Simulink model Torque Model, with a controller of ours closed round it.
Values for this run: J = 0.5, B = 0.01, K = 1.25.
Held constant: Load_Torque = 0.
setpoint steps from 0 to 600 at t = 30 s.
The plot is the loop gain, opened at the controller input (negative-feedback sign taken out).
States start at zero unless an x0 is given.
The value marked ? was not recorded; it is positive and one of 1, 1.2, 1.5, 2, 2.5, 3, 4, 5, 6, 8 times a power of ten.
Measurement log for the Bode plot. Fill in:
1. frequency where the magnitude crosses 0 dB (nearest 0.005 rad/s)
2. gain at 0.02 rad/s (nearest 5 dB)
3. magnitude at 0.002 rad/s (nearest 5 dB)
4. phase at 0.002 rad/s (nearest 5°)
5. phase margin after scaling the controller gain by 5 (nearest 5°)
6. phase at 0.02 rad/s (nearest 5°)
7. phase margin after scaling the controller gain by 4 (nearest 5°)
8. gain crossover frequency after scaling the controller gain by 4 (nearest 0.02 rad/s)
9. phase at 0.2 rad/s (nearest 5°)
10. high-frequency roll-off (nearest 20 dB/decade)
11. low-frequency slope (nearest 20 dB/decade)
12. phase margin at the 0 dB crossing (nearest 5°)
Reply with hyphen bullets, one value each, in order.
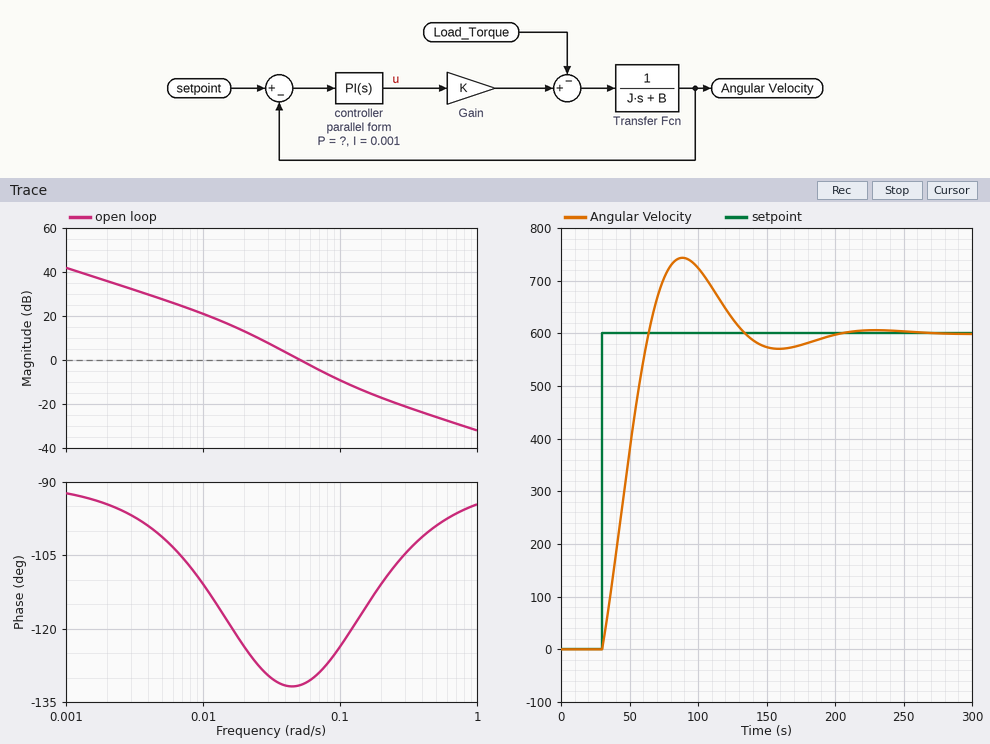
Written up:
- 0.050 rad/s
- 15 dB
- 35 dB
- -95°
- 65°
- -125°
- 60°
- 0.12 rad/s
- -110°
- -20 dB/decade
- -20 dB/decade
- 50°
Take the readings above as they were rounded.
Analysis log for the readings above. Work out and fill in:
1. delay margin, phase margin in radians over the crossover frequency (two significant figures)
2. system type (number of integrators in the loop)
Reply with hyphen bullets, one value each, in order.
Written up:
- 17 s
- 1
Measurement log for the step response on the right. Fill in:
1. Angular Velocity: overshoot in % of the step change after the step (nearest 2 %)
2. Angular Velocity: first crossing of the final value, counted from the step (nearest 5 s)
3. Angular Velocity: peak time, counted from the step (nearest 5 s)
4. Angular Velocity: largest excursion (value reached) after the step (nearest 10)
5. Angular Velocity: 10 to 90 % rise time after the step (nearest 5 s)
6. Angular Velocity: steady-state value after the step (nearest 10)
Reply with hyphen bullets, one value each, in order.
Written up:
- 24 %
- 35 s
- 60 s
- 740
- 25 s
- 600
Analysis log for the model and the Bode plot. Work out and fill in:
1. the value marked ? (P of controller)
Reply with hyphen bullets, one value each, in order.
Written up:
- 0.01
